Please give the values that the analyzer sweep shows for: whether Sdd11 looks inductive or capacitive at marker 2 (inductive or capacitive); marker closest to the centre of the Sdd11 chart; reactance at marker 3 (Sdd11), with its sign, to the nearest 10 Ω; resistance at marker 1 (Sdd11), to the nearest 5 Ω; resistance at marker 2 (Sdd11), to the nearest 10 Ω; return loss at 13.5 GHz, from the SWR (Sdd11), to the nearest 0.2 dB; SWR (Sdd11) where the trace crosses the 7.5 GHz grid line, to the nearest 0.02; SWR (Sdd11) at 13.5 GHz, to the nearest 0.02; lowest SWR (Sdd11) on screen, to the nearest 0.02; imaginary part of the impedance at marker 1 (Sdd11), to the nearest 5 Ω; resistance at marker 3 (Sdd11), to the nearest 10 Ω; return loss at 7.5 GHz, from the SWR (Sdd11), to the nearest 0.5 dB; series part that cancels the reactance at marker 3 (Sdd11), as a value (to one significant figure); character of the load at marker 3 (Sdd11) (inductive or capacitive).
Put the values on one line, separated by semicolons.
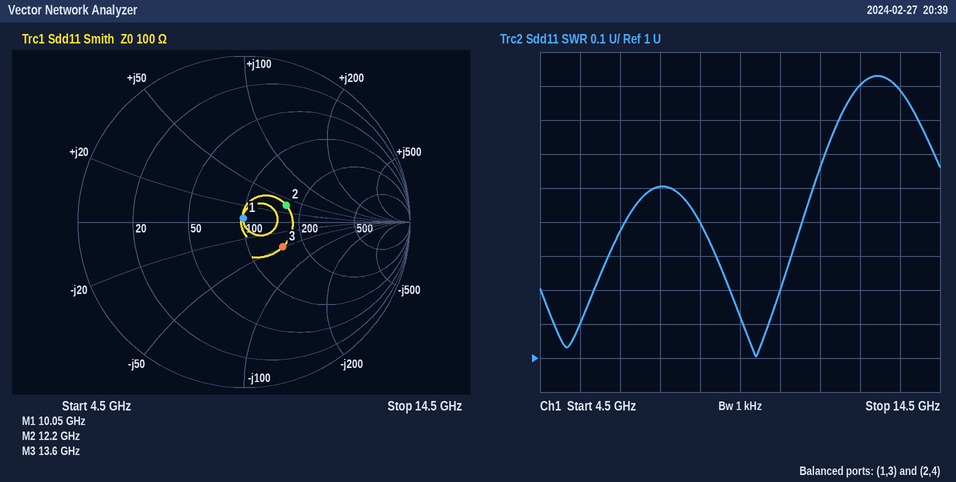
inductive; marker 1; -50 Ω; 100 Ω; 160 Ω; 11.0 dB; 1.50; 1.78; 1.00; +5 Ω; 150 Ω; 14.0 dB; 600 pH; capacitive
